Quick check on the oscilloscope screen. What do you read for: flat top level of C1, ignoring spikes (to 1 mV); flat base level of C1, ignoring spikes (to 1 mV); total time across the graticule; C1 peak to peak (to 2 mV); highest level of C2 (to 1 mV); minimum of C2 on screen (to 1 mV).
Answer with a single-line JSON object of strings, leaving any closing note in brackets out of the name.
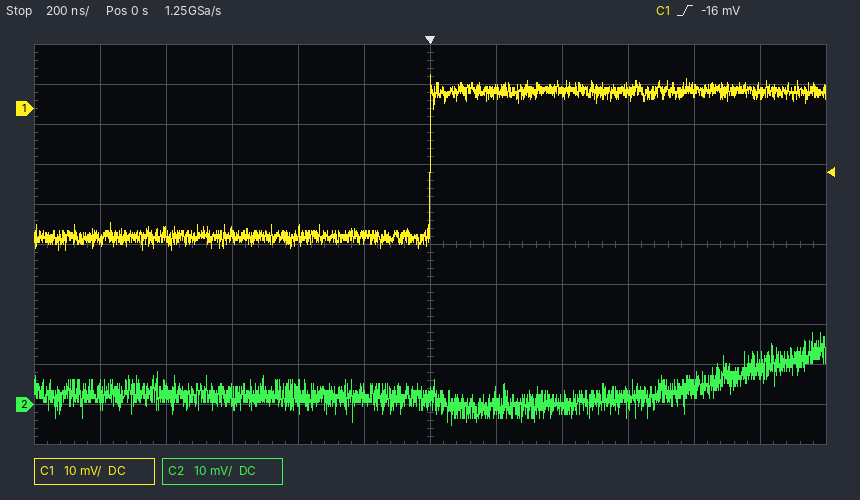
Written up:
{"flat top level of C1, ignoring spikes": "4 mV", "flat base level of C1, ignoring spikes": "-32 mV", "total time across the graticule": "2.4 µs", "C1 peak to peak": "44 mV", "highest level of C2": "18 mV", "minimum of C2 on screen": "-5 mV"}
